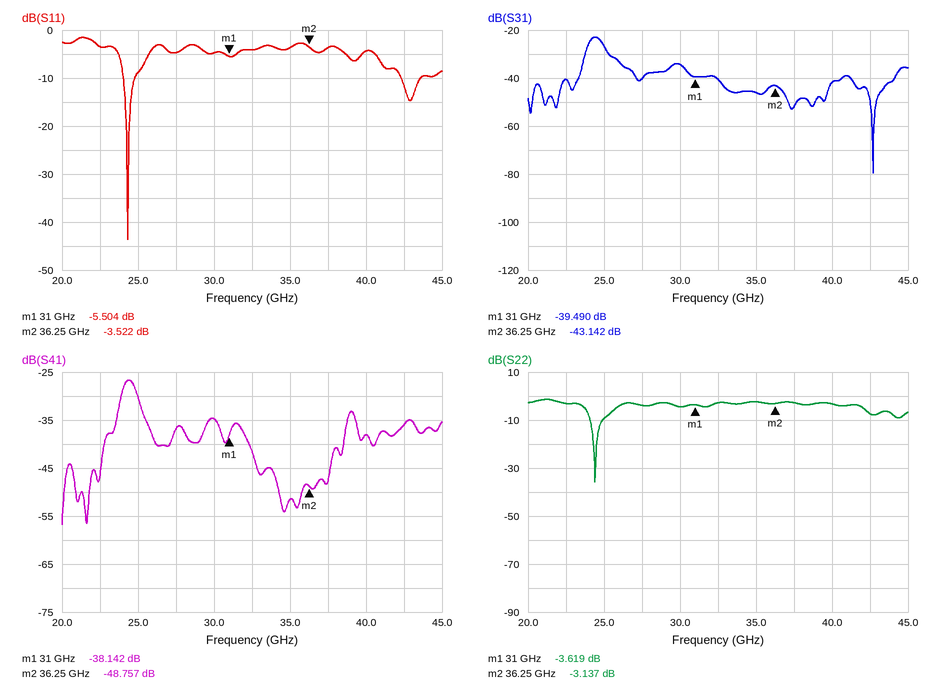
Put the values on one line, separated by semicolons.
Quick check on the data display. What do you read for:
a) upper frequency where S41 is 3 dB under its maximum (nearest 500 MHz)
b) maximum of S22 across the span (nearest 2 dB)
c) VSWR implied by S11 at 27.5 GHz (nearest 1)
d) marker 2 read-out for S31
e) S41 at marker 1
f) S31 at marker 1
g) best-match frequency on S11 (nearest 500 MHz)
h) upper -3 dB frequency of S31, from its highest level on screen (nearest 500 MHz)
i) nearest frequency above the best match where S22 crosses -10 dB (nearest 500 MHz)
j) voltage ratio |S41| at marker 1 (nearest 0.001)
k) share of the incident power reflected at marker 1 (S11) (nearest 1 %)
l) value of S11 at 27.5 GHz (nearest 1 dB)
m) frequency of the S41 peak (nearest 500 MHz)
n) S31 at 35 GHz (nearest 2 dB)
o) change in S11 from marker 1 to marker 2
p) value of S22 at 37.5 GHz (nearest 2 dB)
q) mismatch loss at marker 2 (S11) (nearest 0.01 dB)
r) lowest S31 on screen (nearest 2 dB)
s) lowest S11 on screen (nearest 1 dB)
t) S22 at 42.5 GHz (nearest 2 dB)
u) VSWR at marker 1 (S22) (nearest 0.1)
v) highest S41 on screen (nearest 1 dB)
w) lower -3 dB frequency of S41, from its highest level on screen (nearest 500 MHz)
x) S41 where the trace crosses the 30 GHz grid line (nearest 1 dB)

25.0 GHz; -2 dB; 4; -43.142 dB; -38.142 dB; -39.490 dB; 24.5 GHz; 25.0 GHz; 25.0 GHz; 0.012; 28 %; -5 dB; 24.5 GHz; -46 dB; 1.982 dB; -2 dB; 2.55 dB; -80 dB; -44 dB; -8 dB; 4.9; -27 dB; 24.0 GHz; -35 dB
